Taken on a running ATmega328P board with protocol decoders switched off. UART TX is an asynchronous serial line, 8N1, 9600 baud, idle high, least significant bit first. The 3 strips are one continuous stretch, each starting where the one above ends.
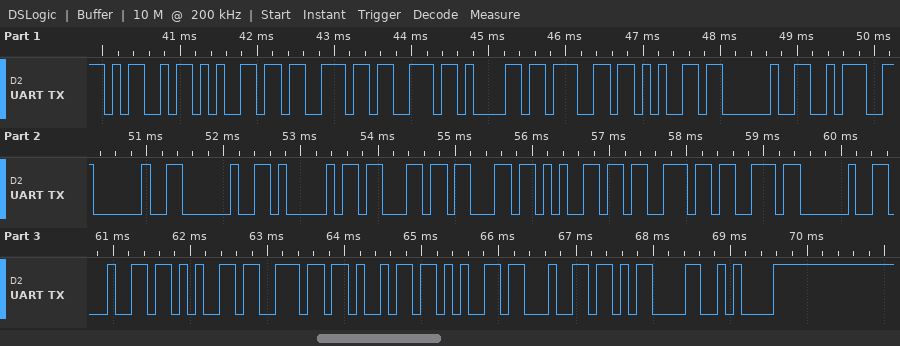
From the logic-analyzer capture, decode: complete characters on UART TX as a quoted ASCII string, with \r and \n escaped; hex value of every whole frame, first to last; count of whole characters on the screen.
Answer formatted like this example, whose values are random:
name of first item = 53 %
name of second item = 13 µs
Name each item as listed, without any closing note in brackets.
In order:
complete characters on UART TX as a quoted ASCII string, with \r and \n escaped = "Message :  Access denied\r\n"
hex value of every whole frame, first to last = 0x4D 0x65 0x73 0x73 0x61 0x67 0x65 0x20 0x3A 0x20 0x20 0x41 0x63 0x63 0x65 0x73 0x73 0x20 0x64 0x65 0x6E 0x69 0x65 0x64 0x0D 0x0A
count of whole characters on the screen = 26
